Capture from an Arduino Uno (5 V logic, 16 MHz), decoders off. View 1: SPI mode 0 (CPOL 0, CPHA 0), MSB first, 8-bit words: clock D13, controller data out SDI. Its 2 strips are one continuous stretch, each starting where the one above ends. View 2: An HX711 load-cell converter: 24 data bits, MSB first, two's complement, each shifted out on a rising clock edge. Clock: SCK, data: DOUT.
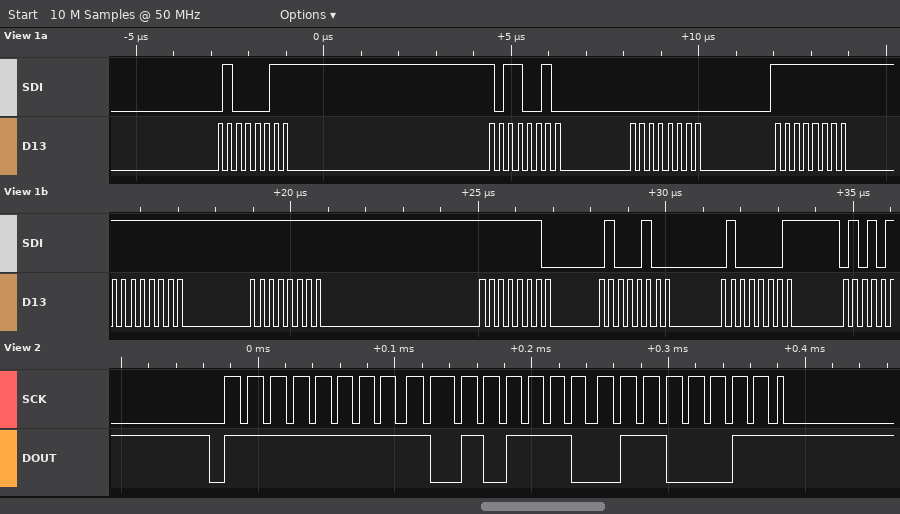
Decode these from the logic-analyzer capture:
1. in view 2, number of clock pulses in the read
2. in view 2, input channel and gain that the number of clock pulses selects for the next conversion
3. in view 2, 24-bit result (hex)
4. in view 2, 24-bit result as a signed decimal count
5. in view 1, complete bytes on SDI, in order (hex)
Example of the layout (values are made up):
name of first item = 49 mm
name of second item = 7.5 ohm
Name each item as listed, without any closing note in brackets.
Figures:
in view 2, number of clock pulses in the read = 25
in view 2, input channel and gain that the number of clock pulses selects for the next conversion = channel A, gain 128
in view 2, 24-bit result = 0xFFAE63
in view 2, 24-bit result as a signed decimal count = -20893
in view 1, complete bytes on SDI, in order = 43 B2 00 FF FF FF FE 44 41
